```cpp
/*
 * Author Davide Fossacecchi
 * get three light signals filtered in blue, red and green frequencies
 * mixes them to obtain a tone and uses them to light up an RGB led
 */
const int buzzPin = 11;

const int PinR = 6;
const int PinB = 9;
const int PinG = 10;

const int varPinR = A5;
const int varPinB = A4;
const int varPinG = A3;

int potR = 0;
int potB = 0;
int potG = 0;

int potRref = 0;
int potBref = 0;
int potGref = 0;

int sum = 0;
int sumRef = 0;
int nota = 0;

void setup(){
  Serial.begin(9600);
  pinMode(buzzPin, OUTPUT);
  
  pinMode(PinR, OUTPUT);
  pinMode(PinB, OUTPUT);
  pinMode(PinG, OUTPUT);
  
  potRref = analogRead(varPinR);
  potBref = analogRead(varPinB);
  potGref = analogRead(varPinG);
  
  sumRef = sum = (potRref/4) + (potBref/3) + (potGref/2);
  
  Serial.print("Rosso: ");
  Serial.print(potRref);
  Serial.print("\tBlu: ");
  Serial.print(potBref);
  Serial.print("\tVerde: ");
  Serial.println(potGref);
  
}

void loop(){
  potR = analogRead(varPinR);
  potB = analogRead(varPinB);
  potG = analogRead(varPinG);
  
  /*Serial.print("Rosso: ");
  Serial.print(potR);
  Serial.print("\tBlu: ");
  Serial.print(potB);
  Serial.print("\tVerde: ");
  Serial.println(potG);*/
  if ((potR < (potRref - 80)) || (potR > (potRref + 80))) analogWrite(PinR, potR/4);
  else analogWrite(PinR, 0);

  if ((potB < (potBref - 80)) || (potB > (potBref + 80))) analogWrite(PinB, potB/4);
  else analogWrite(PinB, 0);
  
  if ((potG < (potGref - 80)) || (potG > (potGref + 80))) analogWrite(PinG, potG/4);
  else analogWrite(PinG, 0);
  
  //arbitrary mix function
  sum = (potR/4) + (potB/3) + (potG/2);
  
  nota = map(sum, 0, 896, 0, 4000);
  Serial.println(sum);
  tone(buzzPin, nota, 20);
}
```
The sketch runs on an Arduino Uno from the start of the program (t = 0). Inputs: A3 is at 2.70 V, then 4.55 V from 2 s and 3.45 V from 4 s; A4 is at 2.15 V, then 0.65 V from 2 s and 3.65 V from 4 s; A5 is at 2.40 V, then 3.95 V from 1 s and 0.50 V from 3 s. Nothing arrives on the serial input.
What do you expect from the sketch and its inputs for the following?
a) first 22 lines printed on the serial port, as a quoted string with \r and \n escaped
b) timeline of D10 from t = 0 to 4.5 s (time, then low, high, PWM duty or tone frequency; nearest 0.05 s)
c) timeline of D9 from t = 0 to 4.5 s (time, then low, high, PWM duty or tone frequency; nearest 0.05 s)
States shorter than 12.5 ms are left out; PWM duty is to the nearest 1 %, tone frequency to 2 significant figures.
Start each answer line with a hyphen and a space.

- "Rosso: 491\tBlu: 440\tVerde: 552\r\n544\r\n544\r\n544\r\n544\r\n544\r\n544\r\n544\r\n544\r\n544\r\n544\r\n544\r\n544\r\n544\r\n544\r\n544\r\n544\r\n544\r\n544\r\n544\r\n544\r\n544\r\n"
- 0 s low; 2 s PWM 91 %; 4 s PWM 69 %
- 0 s low; 2 s PWM 13 %; 4 s PWM 73 %
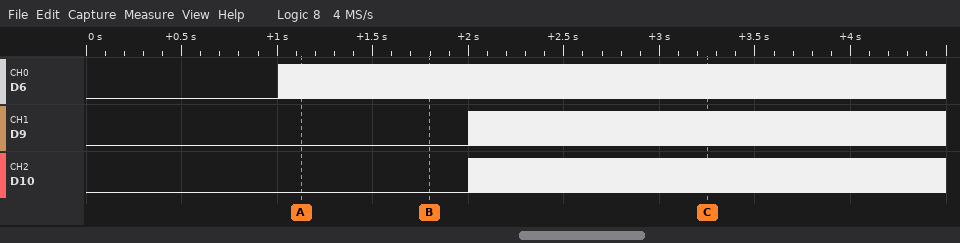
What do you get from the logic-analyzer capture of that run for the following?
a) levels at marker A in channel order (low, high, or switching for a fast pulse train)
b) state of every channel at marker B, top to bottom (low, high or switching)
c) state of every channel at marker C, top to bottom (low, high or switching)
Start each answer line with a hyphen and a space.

- D6 switching, D9 low, D10 low
- D6 switching, D9 low, D10 low
- D6 switching, D9 switching, D10 switching
